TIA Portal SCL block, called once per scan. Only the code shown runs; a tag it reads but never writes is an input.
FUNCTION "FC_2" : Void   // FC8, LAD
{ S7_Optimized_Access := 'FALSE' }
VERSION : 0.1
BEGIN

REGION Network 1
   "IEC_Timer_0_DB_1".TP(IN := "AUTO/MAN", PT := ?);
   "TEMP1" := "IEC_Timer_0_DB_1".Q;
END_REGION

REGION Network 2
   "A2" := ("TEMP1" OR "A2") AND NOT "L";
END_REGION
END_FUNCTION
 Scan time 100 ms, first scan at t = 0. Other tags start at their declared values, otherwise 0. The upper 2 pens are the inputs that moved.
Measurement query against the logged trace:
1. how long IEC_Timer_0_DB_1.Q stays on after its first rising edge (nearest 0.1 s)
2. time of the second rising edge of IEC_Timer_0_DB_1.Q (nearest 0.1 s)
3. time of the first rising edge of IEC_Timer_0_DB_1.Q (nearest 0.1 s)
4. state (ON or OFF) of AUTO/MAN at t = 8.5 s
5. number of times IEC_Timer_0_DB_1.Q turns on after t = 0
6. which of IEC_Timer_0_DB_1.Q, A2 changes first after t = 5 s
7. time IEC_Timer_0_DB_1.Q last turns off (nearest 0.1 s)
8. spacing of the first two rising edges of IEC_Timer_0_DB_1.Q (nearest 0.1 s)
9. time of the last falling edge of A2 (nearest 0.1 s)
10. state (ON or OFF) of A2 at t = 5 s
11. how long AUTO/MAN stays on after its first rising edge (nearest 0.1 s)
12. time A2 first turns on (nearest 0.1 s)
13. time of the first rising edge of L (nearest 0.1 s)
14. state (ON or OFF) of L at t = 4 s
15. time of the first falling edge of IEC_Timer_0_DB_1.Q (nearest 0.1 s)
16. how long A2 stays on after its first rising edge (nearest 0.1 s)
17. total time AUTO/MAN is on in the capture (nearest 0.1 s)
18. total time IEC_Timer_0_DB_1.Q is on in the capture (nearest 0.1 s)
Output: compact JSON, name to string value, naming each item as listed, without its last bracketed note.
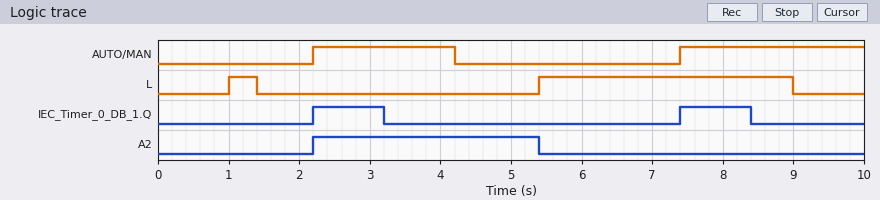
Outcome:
{"how long IEC_Timer_0_DB_1.Q stays on after its first rising edge": "1.0 s", "time of the second rising edge of IEC_Timer_0_DB_1.Q": "7.4 s", "time of the first rising edge of IEC_Timer_0_DB_1.Q": "2.2 s", "state (ON or OFF) of AUTO/MAN at t = 8.5 s": "ON", "number of times IEC_Timer_0_DB_1.Q turns on after t = 0": "2", "which of IEC_Timer_0_DB_1.Q, A2 changes first after t = 5 s": "A2", "time IEC_Timer_0_DB_1.Q last turns off": "8.4 s", "spacing of the first two rising edges of IEC_Timer_0_DB_1.Q": "5.2 s", "time of the last falling edge of A2": "5.4 s", "state (ON or OFF) of A2 at t = 5 s": "ON", "how long AUTO/MAN stays on after its first rising edge": "2.0 s", "time A2 first turns on": "2.2 s", "time of the first rising edge of L": "1.0 s", "state (ON or OFF) of L at t = 4 s": "OFF", "time of the first falling edge of IEC_Timer_0_DB_1.Q": "3.2 s", "how long A2 stays on after its first rising edge": "3.2 s", "total time AUTO/MAN is on in the capture": "4.6 s", "total time IEC_Timer_0_DB_1.Q is on in the capture": "2.0 s"}
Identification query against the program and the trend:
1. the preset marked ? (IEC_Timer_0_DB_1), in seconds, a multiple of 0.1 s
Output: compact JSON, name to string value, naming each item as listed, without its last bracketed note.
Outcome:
{"the preset marked ? (IEC_Timer_0_DB_1), in seconds, a multiple of 0.1 s": "1.0 s"}
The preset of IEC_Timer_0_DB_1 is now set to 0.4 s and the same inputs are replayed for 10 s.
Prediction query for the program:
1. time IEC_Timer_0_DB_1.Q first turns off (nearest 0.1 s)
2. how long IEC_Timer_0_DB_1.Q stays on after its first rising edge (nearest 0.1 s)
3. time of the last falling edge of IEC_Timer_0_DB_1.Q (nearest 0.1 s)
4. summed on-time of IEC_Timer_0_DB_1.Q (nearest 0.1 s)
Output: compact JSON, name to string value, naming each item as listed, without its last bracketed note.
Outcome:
{"time IEC_Timer_0_DB_1.Q first turns off": "2.6 s", "how long IEC_Timer_0_DB_1.Q stays on after its first rising edge": "0.4 s", "time of the last falling edge of IEC_Timer_0_DB_1.Q": "7.8 s", "summed on-time of IEC_Timer_0_DB_1.Q": "0.8 s"}
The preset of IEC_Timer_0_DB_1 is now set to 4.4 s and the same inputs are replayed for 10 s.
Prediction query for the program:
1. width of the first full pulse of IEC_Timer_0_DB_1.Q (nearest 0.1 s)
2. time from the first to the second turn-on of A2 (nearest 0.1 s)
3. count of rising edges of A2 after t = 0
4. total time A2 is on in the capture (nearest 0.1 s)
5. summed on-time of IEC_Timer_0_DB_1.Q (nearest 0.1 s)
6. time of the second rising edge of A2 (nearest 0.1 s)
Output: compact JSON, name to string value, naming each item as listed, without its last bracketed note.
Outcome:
{"width of the first full pulse of IEC_Timer_0_DB_1.Q": "4.4 s", "time from the first to the second turn-on of A2": "6.8 s", "count of rising edges of A2 after t = 0": "2", "total time A2 is on in the capture": "4.2 s", "summed on-time of IEC_Timer_0_DB_1.Q": "7.0 s", "time of the second rising edge of A2": "9.0 s"}
